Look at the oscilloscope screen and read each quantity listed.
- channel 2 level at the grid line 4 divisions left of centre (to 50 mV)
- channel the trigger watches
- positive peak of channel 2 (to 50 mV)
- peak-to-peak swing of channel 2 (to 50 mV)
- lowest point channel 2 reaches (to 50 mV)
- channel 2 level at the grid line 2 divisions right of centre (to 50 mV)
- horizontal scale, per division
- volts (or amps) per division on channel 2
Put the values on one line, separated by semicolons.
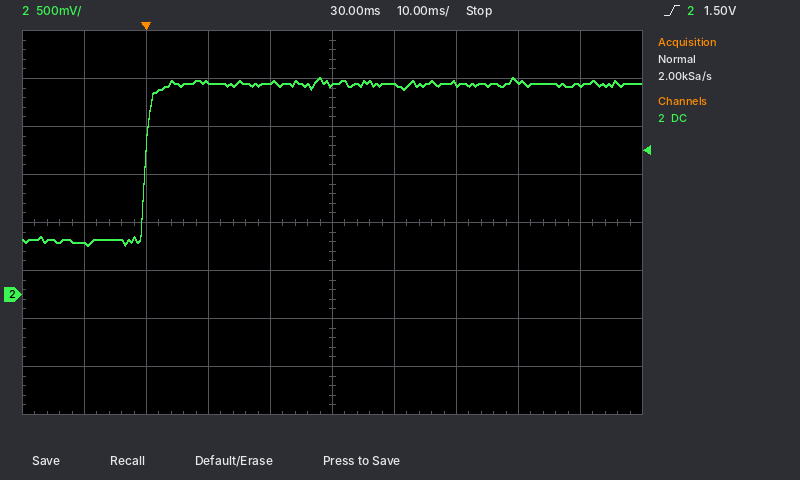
550 mV; channel 2; 2.25 V; 1.75 V; 500 mV; 2.20 V; 10 ms; 500 mV
